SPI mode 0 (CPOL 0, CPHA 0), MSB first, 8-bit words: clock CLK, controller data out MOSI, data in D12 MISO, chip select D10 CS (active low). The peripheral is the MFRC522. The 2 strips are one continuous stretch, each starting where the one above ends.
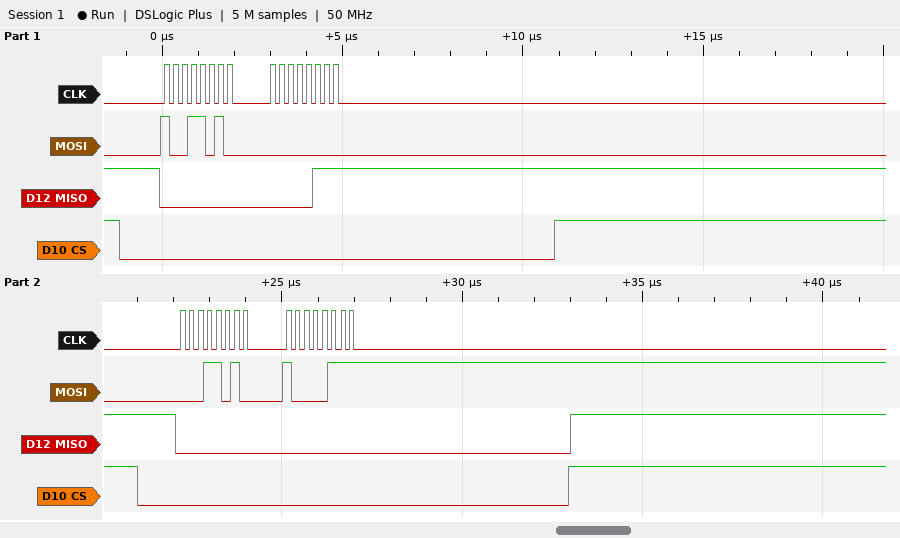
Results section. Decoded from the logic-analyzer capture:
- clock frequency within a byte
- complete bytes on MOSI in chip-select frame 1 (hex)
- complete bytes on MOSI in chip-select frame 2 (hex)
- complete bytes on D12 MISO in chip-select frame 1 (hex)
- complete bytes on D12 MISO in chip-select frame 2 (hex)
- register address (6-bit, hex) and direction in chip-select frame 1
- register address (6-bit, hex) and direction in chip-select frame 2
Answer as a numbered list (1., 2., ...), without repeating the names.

1. 4 MHz
2. 9A 00
3. 1A 87
4. 00 07
5. 00 00
6. 0x0D read
7. 0x0D write
